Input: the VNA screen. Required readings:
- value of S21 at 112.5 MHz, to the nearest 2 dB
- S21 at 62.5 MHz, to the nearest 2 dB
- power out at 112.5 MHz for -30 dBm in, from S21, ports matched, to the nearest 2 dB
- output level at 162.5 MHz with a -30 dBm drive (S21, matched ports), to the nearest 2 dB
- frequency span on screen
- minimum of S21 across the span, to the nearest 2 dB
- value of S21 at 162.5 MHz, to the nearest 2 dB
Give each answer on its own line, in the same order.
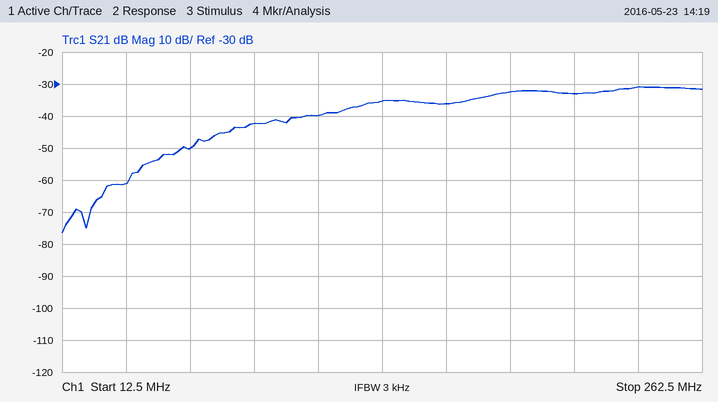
-40 dB
-50 dB
-70 dBm
-66 dBm
250 MHz
-76 dB
-36 dB
